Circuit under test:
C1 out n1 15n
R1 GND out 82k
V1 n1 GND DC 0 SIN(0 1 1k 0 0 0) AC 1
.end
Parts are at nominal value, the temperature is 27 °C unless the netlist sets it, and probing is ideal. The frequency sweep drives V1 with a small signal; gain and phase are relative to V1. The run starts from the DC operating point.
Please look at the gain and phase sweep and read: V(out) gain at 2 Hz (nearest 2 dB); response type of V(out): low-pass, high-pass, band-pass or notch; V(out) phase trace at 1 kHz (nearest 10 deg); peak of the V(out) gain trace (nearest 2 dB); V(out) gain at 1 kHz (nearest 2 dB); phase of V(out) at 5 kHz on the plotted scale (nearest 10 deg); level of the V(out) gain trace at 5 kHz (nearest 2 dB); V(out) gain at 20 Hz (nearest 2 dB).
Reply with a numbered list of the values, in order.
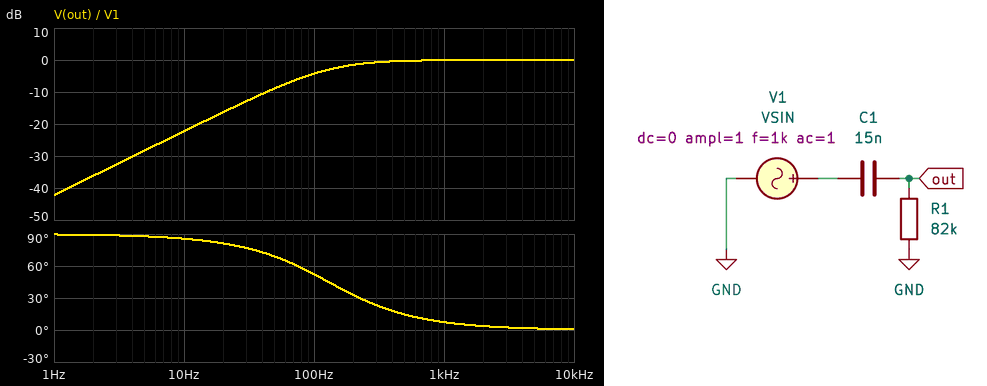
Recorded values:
1. -36 dB
2. high-pass
3. 10 deg
4. 0 dB
5. 0 dB
6. 0 deg
7. 0 dB
8. -16 dB
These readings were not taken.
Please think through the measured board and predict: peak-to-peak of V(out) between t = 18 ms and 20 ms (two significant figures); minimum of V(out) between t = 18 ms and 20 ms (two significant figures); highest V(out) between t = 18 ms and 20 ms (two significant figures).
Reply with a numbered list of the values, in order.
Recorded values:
1. 2.0 V
2. -990 mV
3. 990 mV
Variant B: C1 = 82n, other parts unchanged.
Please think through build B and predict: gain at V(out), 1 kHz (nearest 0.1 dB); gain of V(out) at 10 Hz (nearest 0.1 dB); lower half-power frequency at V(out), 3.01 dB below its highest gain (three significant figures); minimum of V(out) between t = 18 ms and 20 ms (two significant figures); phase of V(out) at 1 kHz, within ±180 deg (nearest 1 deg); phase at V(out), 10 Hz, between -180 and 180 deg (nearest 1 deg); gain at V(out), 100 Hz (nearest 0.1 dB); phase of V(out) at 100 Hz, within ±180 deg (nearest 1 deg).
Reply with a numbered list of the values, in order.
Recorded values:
1. 0 dB
2. -8.2 dB
3. 23.7 Hz
4. -1.0 V
5. 1 deg
6. 67 deg
7. -0.2 dB
8. 13 deg
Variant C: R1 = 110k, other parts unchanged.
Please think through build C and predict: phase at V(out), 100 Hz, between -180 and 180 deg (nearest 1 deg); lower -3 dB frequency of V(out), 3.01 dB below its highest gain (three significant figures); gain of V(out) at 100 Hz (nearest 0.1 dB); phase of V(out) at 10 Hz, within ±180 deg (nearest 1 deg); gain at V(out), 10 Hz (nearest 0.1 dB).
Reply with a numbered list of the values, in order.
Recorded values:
1. 44 deg
2. 96.5 Hz
3. -2.9 dB
4. 84 deg
5. -19.7 dB
